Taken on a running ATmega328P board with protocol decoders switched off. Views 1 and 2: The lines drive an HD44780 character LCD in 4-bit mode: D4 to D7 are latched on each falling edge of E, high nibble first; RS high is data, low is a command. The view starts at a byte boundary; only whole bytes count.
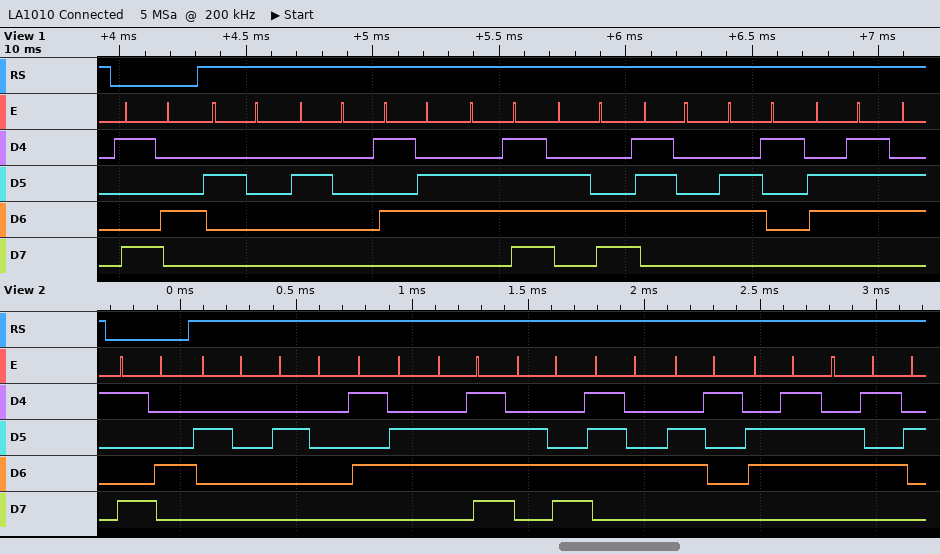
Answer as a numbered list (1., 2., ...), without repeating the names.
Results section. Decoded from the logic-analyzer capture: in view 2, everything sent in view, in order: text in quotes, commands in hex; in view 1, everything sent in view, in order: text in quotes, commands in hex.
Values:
1. 0x94 "  Voltage"
2. 0x94 "  Voltag"
